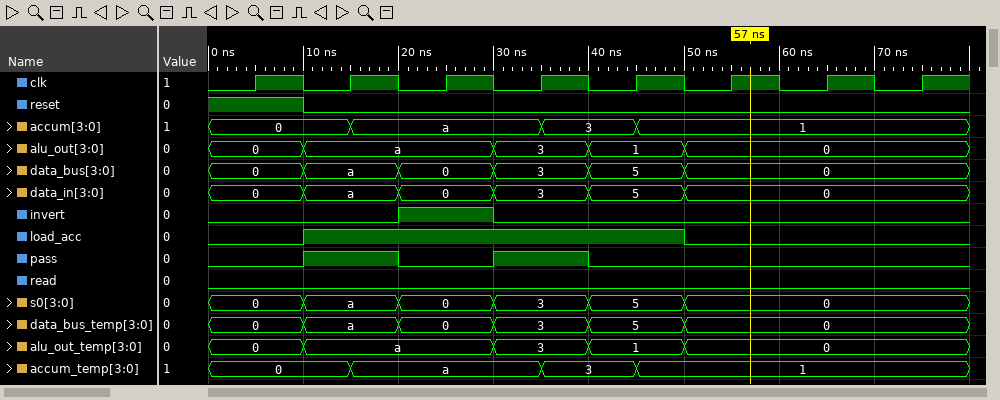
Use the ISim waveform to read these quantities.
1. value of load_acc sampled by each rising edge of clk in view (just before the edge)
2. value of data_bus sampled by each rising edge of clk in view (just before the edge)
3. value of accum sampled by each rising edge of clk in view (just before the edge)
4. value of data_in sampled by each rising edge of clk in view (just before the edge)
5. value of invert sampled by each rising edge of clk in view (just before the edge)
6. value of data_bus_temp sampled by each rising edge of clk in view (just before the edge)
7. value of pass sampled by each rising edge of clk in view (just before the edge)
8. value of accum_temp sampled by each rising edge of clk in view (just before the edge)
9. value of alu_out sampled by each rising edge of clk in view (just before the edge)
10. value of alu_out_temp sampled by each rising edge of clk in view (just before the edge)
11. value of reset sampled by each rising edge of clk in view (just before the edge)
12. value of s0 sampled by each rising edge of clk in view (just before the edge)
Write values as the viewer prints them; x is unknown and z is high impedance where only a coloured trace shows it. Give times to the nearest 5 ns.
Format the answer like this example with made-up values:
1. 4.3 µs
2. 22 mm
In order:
1. 0 1 1 1 1 0 0 0
2. 0, a, 0, 3, 5, 0, 0, 0
3. 0, 0, a, a, 3, 1, 1, 1
4. 0, a, 0, 3, 5, 0, 0, 0
5. 0 0 1 0 0 0 0 0
6. 0, a, 0, 3, 5, 0, 0, 0
7. 0 1 0 1 0 0 0 0
8. 0, 0, a, a, 3, 1, 1, 1
9. 0, a, a, 3, 1, 0, 0, 0
10. 0, a, a, 3, 1, 0, 0, 0
11. 1 0 0 0 0 0 0 0
12. 0, a, 0, 3, 5, 0, 0, 0
